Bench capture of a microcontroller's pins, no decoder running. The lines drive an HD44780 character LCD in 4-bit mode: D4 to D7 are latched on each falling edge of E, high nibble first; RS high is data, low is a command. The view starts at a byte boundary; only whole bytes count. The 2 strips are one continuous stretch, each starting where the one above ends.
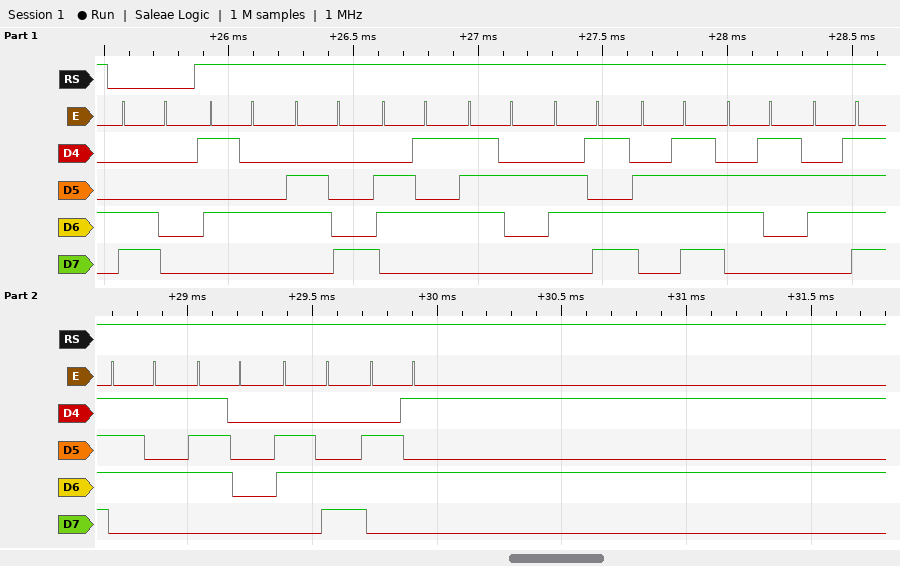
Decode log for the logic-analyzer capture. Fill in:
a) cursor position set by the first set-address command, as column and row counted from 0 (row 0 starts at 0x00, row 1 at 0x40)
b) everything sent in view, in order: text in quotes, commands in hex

column 0, row 1
0xC0 "Thermocouple"
